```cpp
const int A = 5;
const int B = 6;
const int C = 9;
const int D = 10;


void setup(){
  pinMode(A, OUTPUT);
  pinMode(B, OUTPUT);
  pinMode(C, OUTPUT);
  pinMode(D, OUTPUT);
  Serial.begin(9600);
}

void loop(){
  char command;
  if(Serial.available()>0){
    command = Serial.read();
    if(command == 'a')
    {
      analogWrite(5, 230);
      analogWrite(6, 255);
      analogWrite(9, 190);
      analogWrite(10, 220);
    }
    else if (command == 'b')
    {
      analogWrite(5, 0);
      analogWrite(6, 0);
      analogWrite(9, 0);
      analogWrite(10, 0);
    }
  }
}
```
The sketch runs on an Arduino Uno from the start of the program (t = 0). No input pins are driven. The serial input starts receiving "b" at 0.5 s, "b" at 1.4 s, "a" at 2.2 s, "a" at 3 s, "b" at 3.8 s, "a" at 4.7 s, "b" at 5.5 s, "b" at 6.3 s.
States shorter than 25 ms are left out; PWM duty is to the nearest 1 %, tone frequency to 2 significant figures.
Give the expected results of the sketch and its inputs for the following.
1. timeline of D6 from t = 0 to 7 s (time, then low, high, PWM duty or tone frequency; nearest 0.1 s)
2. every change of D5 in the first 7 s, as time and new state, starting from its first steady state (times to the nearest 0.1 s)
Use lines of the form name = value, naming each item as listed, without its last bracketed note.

timeline of D6 from t = 0 to 7 s = 0 s low; 2.2 s high; 3.8 s low; 4.7 s high; 5.5 s low
every change of D5 in the first 7 s, as time and new state, starting from its first steady state = 0 s low; 2.2 s PWM 90 %; 3.8 s low; 4.7 s PWM 90 %; 5.5 s low
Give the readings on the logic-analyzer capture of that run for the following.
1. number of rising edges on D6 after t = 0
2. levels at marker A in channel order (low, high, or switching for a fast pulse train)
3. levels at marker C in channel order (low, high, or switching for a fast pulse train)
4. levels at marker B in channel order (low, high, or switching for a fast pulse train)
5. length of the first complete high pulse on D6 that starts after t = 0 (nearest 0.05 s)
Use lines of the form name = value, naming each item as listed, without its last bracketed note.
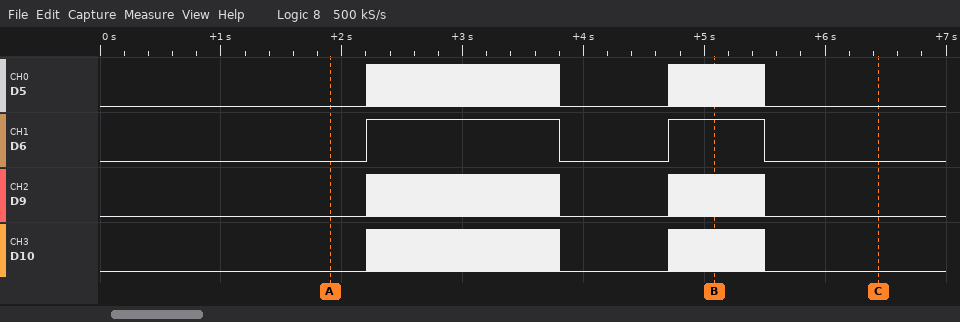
number of rising edges on D6 after t = 0 = 2
levels at marker A in channel order = D5 low, D6 low, D9 low, D10 low
levels at marker C in channel order = D5 low, D6 low, D9 low, D10 low
levels at marker B in channel order = D5 switching, D6 high, D9 switching, D10 switching
length of the first complete high pulse on D6 that starts after t = 0 = 1.60 s
